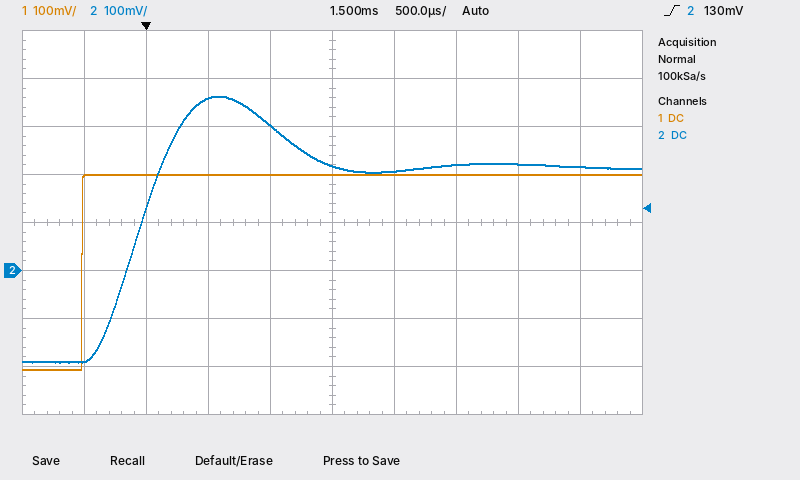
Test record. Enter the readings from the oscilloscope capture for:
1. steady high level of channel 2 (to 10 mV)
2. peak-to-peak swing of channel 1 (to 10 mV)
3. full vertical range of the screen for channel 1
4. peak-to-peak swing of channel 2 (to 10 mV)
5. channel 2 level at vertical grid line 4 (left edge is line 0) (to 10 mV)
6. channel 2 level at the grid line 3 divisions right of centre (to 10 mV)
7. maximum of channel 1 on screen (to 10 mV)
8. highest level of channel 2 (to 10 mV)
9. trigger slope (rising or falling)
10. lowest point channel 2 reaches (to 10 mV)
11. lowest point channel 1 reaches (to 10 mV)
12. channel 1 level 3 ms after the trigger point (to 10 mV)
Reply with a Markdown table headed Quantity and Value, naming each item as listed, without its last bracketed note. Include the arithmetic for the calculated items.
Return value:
| Quantity | Value |
|---|---|
| steady high level of channel 2 | 220 mV |
| peak-to-peak swing of channel 1 | 200 mV − (-210 mV) = 410 mV |
| full vertical range of the screen for channel 1 | 800 mV |
| peak-to-peak swing of channel 2 | 360 mV − (-190 mV) = 550 mV |
| channel 2 level at vertical grid line 4 (left edge is line 0) | 300 mV |
| channel 2 level at the grid line 3 divisions right of centre | 220 mV |
| maximum of channel 1 on screen | 200 mV |
| highest level of channel 2 | 360 mV |
| trigger slope | rising |
| lowest point channel 2 reaches | -190 mV |
| lowest point channel 1 reaches | -210 mV |
| channel 1 level 3 ms after the trigger point | 200 mV |
